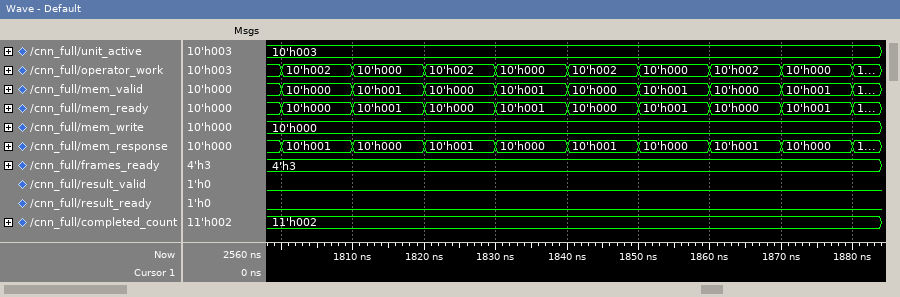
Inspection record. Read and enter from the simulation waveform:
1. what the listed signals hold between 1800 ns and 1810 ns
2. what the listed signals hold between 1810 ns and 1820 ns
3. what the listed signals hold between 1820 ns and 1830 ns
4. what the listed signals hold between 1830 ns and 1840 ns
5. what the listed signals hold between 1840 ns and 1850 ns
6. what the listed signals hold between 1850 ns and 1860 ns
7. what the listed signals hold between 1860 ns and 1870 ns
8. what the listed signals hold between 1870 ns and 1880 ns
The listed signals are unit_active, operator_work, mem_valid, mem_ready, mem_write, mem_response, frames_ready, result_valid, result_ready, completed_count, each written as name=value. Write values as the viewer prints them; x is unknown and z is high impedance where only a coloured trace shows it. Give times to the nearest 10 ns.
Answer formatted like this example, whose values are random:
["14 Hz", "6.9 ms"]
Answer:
["unit_active=10'h003, operator_work=10'h002, mem_valid=10'h000, mem_ready=10'h000, mem_write=10'h000, mem_response=10'h001, frames_ready=4'h3, result_valid=0, result_ready=0, completed_count=11'h002", "unit_active=10'h003, operator_work=10'h000, mem_valid=10'h001, mem_ready=10'h001, mem_write=10'h000, mem_response=10'h000, frames_ready=4'h3, result_valid=0, result_ready=0, completed_count=11'h002", "unit_active=10'h003, operator_work=10'h002, mem_valid=10'h000, mem_ready=10'h000, mem_write=10'h000, mem_response=10'h001, frames_ready=4'h3, result_valid=0, result_ready=0, completed_count=11'h002", "unit_active=10'h003, operator_work=10'h000, mem_valid=10'h001, mem_ready=10'h001, mem_write=10'h000, mem_response=10'h000, frames_ready=4'h3, result_valid=0, result_ready=0, completed_count=11'h002", "unit_active=10'h003, operator_work=10'h002, mem_valid=10'h000, mem_ready=10'h000, mem_write=10'h000, mem_response=10'h001, frames_ready=4'h3, result_valid=0, result_ready=0, completed_count=11'h002", "unit_active=10'h003, operator_work=10'h000, mem_valid=10'h001, mem_ready=10'h001, mem_write=10'h000, mem_response=10'h000, frames_ready=4'h3, result_valid=0, result_ready=0, completed_count=11'h002", "unit_active=10'h003, operator_work=10'h002, mem_valid=10'h000, mem_ready=10'h000, mem_write=10'h000, mem_response=10'h001, frames_ready=4'h3, result_valid=0, result_ready=0, completed_count=11'h002", "unit_active=10'h003, operator_work=10'h000, mem_valid=10'h001, mem_ready=10'h001, mem_write=10'h000, mem_response=10'h000, frames_ready=4'h3, result_valid=0, result_ready=0, completed_count=11'h002"]
